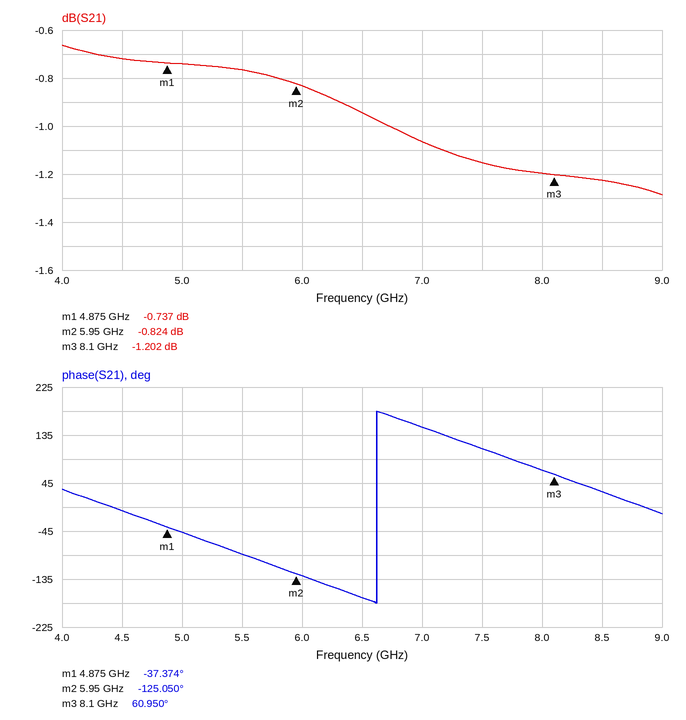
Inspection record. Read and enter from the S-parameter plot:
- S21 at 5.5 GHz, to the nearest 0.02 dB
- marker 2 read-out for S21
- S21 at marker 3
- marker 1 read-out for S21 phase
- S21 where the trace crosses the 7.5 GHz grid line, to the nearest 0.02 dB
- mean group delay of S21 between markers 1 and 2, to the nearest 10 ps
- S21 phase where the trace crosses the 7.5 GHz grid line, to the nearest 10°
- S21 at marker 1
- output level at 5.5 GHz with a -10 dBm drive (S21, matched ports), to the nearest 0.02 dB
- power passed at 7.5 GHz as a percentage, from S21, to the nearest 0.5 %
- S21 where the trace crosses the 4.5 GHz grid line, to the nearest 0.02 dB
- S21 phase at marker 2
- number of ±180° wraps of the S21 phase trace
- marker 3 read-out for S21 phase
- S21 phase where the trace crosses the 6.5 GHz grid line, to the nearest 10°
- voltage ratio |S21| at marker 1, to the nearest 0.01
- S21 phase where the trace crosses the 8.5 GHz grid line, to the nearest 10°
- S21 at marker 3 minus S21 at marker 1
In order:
-0.76 dB
-0.824 dB
-1.202 dB
-37.374°
-1.16 dB
230 ps
110°
-0.737 dB
-10.76 dBm
76.5 %
-0.72 dB
-125.050°
1
60.950°
-170°
0.92
30°
-0.465 dB
